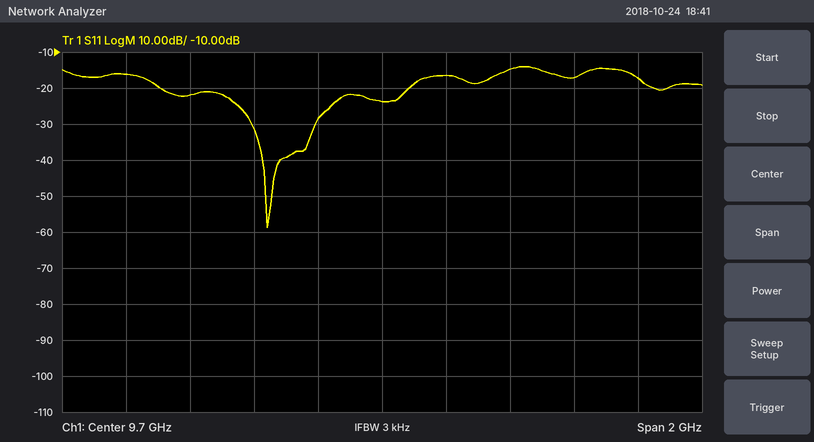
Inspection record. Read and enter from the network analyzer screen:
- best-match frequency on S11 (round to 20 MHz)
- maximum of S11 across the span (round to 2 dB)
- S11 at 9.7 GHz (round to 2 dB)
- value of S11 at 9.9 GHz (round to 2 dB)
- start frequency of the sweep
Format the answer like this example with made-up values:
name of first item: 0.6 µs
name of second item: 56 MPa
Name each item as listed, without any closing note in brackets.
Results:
best-match frequency on S11: 9.34 GHz
maximum of S11 across the span: -14 dB
S11 at 9.7 GHz: -24 dB
value of S11 at 9.9 GHz: -16 dB
start frequency of the sweep: 8.7 GHz
